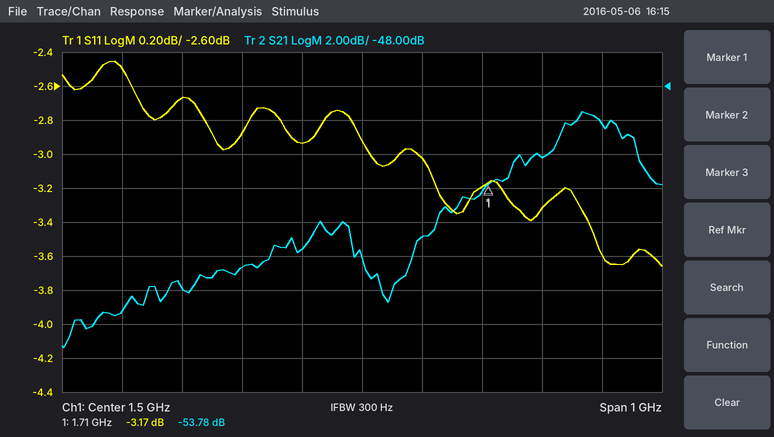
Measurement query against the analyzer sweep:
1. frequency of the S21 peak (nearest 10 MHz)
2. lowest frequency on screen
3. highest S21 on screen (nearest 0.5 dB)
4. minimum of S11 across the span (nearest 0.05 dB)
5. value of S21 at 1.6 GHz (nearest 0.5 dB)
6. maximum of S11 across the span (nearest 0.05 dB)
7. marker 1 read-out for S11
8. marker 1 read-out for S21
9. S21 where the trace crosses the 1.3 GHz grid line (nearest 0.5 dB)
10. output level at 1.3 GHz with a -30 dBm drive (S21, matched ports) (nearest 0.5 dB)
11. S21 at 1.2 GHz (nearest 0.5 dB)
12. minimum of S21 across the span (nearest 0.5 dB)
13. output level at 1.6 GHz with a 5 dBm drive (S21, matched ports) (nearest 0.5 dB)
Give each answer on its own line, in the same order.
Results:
1.87 GHz
1 GHz
-49.5 dB
-3.65 dB
-57.0 dB
-2.45 dB
-3.17 dB
-53.78 dB
-58.5 dB
-88.5 dBm
-60.0 dB
-63.5 dB
-52.0 dBm
